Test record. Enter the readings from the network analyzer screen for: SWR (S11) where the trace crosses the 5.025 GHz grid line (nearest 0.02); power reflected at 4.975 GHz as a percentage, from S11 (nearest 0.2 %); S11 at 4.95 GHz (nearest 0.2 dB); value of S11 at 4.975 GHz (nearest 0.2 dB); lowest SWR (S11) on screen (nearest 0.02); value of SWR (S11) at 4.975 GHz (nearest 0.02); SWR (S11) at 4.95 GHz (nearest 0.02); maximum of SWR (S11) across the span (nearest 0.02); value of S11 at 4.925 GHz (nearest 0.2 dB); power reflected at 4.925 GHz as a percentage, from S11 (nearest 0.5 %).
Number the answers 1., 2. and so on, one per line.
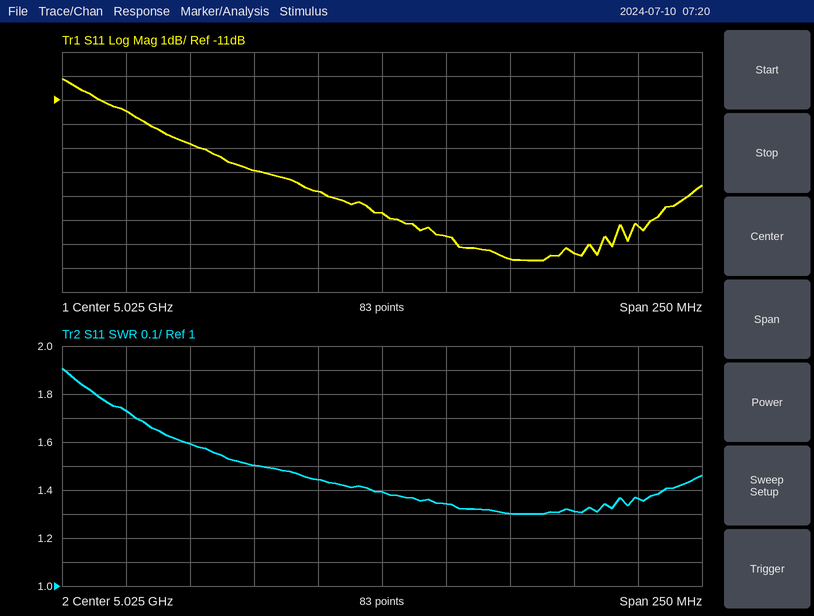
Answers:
1. 1.40
2. 4.0 %
3. -12.8 dB
4. -14.0 dB
5. 1.30
6. 1.50
7. 1.60
8. 1.90
9. -11.4 dB
10. 7.0 %
